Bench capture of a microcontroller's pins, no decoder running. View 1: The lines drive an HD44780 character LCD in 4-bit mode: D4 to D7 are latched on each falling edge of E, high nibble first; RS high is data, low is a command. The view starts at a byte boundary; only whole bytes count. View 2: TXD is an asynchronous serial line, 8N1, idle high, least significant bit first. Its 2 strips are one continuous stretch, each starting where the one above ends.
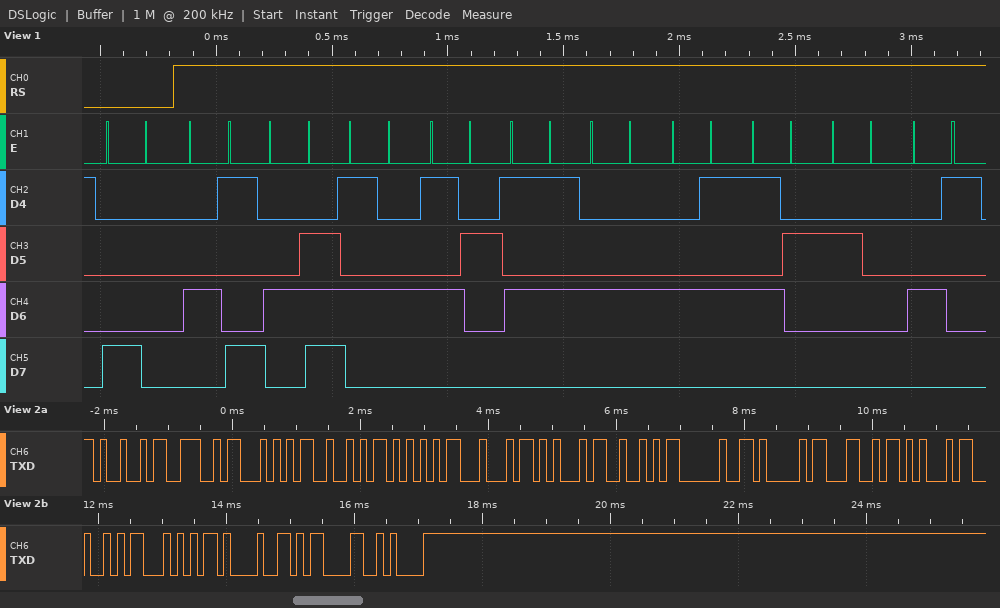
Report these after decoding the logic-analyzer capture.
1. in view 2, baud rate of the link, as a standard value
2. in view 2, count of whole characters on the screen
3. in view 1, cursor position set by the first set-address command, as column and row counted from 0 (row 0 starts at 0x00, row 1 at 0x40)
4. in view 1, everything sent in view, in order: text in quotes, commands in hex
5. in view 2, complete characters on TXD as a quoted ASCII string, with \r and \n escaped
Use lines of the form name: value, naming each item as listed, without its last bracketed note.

in view 2, baud rate of the link, as a standard value: 9600 baud
in view 2, count of whole characters on the screen: 17
in view 1, cursor position set by the first set-address command, as column and row counted from 0: column 0, row 0
in view 1, everything sent in view, in order: text in quotes, commands in hex: 0x80 "INTRUDER A"
in view 2, complete characters on TXD as a quoted ASCII string, with \r and \n escaped: "INTRUDER ALERT!\r\n"
